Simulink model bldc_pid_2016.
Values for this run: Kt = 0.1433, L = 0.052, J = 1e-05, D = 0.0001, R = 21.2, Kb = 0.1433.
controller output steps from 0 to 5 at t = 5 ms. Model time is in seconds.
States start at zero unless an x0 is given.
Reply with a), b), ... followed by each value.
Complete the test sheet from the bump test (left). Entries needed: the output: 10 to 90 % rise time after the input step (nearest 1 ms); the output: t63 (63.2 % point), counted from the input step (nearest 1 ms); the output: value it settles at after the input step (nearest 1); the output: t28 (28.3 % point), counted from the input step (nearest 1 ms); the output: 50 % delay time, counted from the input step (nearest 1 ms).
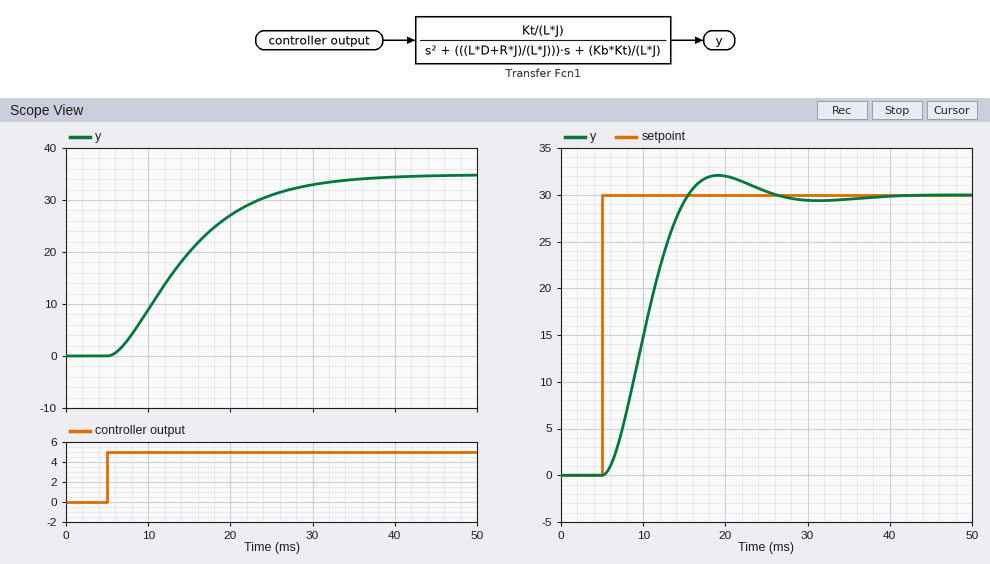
a) 18 ms
b) 11 ms
c) 35
d) 5 ms
e) 9 ms
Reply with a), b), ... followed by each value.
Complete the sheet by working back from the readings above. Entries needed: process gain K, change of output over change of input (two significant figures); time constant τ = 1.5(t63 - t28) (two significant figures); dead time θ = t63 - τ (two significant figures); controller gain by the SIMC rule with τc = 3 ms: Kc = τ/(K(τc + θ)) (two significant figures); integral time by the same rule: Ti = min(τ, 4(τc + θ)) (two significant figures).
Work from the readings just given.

a) 7.0
b) 9.0 ms
c) 2.0 ms
d) 0.26
e) 9.0 ms
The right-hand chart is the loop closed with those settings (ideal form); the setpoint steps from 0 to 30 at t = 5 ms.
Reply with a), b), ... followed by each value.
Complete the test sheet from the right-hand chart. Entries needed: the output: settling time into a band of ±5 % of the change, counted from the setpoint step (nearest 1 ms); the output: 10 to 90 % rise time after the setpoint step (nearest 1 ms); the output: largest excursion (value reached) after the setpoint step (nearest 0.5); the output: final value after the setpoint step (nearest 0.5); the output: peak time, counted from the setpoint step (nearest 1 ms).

a) 17 ms
b) 7 ms
c) 32.0
d) 30.0
e) 14 ms
